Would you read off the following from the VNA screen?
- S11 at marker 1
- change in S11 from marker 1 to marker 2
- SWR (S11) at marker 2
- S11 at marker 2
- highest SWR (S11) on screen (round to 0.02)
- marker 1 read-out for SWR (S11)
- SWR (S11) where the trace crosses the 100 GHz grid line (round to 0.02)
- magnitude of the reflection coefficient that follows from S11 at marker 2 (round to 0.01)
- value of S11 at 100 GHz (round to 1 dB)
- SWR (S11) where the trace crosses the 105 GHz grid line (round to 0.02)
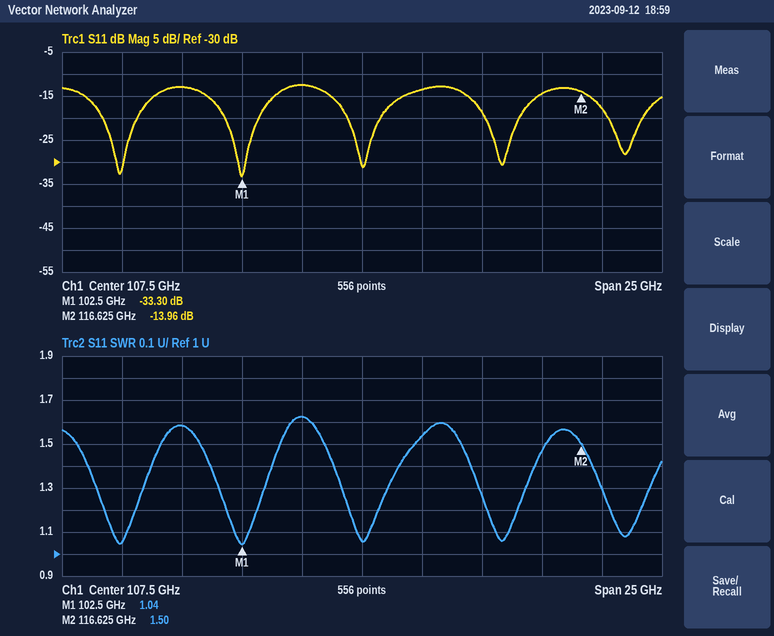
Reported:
-33.30 dB
19.34 dB
1.50
-13.96 dB
1.62
1.04
1.58
0.20
-13 dB
1.62
